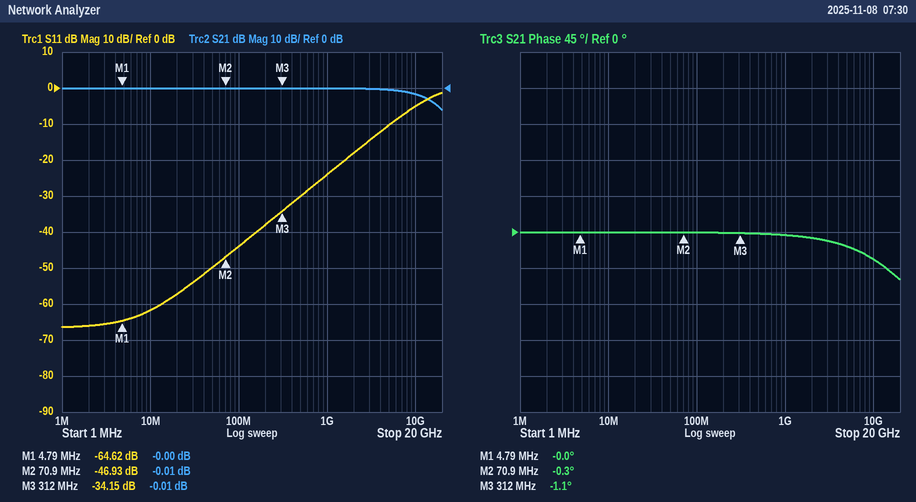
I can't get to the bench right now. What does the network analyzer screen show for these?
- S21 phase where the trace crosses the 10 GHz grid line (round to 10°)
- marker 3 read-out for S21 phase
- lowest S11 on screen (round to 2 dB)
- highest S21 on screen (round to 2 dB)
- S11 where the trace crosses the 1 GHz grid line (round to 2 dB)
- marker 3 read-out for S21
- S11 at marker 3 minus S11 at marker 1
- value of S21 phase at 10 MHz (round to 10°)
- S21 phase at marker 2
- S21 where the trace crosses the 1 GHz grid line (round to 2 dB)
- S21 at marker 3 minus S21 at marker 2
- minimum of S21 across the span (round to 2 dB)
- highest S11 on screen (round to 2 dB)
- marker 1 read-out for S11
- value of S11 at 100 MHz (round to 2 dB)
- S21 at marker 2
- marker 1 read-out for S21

-30°
-1.1°
-66 dB
0 dB
-24 dB
-0.01 dB
30.47 dB
0°
-0.3°
0 dB
0.00 dB
-6 dB
-2 dB
-64.62 dB
-44 dB
-0.01 dB
-0.00 dB
